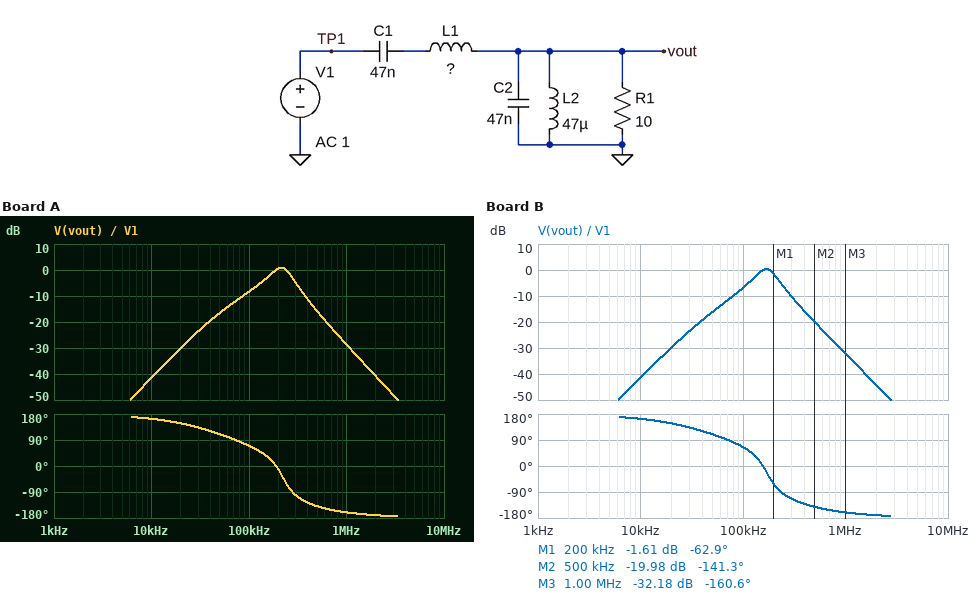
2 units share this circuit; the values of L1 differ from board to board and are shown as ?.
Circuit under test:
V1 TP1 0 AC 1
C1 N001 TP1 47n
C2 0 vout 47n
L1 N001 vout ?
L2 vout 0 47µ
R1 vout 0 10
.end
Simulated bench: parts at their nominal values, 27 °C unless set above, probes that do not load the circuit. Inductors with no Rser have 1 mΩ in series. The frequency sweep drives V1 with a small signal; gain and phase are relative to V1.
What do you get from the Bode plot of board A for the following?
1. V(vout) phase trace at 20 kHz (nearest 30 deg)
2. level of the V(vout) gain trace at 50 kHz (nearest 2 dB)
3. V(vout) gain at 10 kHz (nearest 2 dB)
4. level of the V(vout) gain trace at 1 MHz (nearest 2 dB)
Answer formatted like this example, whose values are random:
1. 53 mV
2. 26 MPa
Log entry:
1. 150 deg
2. -16 dB
3. -42 dB
4. -28 dB
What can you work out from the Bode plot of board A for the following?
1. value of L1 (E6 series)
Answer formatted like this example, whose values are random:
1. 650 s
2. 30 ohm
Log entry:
1. 15 µH
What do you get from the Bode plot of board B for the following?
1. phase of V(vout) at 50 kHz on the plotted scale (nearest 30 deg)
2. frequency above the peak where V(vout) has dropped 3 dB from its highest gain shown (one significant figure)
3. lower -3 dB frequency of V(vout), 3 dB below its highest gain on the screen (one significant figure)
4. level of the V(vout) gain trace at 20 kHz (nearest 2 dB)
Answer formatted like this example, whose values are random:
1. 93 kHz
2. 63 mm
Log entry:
1. 120 deg
2. 200 kHz
3. 100 kHz
4. -30 dB
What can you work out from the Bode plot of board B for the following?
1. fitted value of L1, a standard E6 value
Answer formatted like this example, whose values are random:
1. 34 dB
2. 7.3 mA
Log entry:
1. 22 µH
